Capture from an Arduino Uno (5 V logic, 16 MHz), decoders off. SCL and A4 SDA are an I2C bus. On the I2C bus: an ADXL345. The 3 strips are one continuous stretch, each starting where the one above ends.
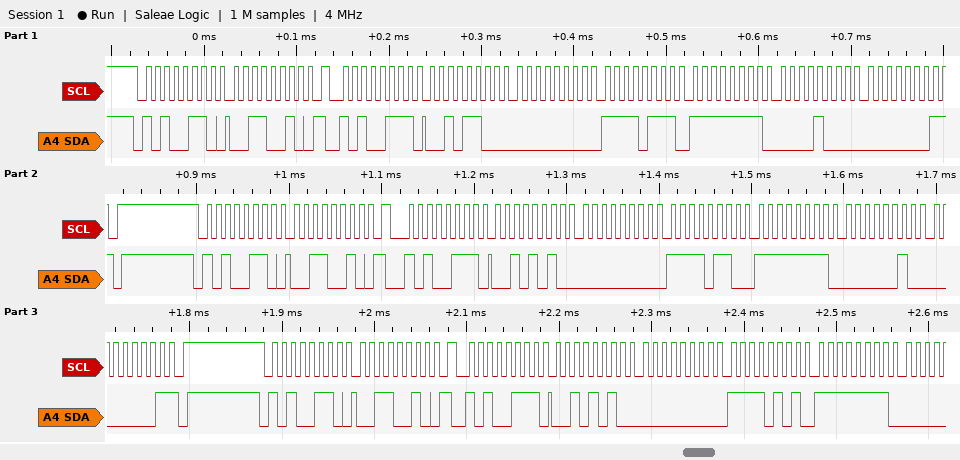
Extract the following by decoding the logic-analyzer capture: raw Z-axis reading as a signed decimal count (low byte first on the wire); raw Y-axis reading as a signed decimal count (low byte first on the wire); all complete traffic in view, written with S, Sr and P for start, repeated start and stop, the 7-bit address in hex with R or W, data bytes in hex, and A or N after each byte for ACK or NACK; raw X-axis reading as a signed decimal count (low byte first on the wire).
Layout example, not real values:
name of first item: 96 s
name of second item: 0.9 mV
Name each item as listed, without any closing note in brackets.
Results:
raw Z-axis reading as a signed decimal count: 264
raw Y-axis reading as a signed decimal count: -9
all complete traffic in view, written with S, Sr and P for start, repeated start and stop, the 7-bit address in hex with R or W, data bytes in hex, and A or N after each byte for ACK or NACK: S 53W A 32 A Sr 53R A 2C A 00 A F7 A FF A 08 A 01 N P S 53W A 32 A Sr 53R A 2A A 00 A F6 A FF A 02 A 01 N P S 53W A 32 A Sr 53R A 2A A 00 A F5 A FF A
raw X-axis reading as a signed decimal count: 44
